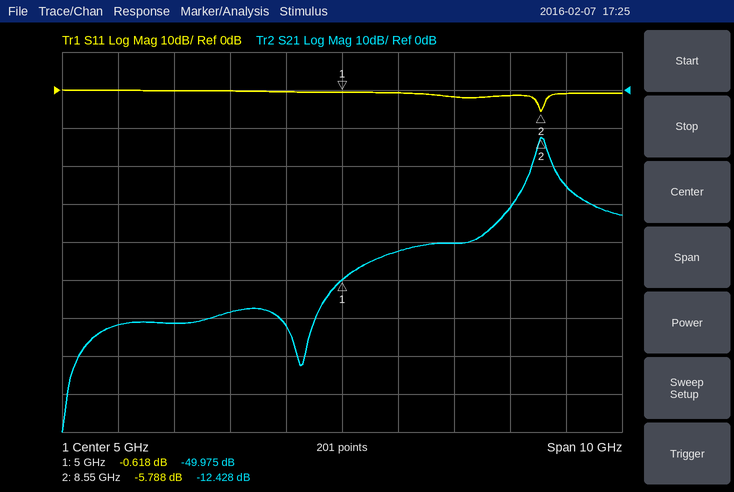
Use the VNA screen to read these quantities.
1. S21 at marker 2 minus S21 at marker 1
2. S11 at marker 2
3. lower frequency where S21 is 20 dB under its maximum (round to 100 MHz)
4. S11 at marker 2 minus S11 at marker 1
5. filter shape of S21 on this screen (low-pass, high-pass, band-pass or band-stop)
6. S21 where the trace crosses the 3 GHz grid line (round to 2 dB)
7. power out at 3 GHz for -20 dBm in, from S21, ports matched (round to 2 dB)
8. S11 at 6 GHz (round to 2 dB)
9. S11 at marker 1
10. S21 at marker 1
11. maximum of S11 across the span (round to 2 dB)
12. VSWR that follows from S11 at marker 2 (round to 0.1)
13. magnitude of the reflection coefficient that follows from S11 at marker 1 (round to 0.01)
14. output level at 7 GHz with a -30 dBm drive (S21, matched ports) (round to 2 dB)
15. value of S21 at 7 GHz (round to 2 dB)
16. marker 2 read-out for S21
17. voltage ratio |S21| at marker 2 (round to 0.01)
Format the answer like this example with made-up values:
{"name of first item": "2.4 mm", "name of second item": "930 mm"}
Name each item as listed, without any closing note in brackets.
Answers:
{"S21 at marker 2 minus S21 at marker 1": "37.547 dB", "S11 at marker 2": "-5.788 dB", "lower frequency where S21 is 20 dB under its maximum": "7.9 GHz", "S11 at marker 2 minus S11 at marker 1": "-5.170 dB", "filter shape of S21 on this screen": "band-pass", "S21 where the trace crosses the 3 GHz grid line": "-58 dB", "power out at 3 GHz for -20 dBm in, from S21, ports matched": "-78 dBm", "S11 at 6 GHz": "0 dB", "S11 at marker 1": "-0.618 dB", "S21 at marker 1": "-49.975 dB", "maximum of S11 across the span": "0 dB", "VSWR that follows from S11 at marker 2": "3.1", "magnitude of the reflection coefficient that follows from S11 at marker 1": "0.93", "output level at 7 GHz with a -30 dBm drive (S21, matched ports)": "-70 dBm", "value of S21 at 7 GHz": "-40 dB", "marker 2 read-out for S21": "-12.428 dB", "voltage ratio |S21| at marker 2": "0.24"}
